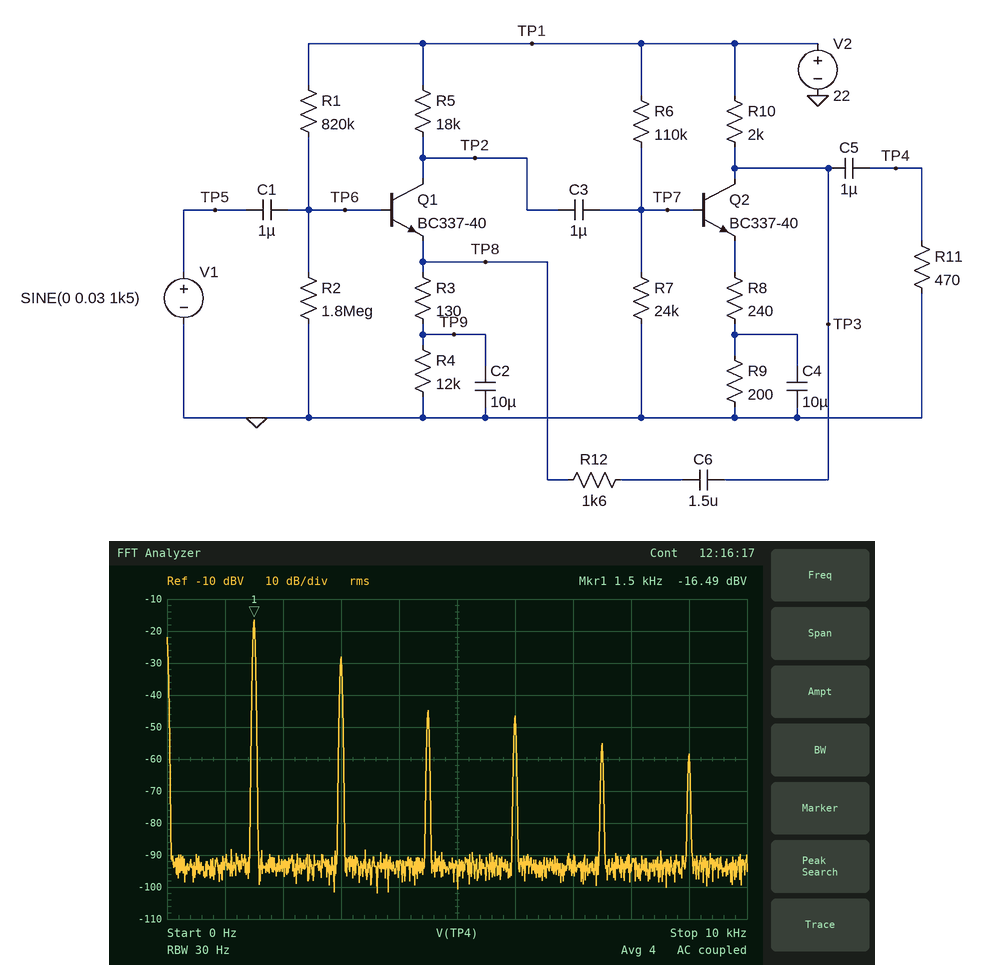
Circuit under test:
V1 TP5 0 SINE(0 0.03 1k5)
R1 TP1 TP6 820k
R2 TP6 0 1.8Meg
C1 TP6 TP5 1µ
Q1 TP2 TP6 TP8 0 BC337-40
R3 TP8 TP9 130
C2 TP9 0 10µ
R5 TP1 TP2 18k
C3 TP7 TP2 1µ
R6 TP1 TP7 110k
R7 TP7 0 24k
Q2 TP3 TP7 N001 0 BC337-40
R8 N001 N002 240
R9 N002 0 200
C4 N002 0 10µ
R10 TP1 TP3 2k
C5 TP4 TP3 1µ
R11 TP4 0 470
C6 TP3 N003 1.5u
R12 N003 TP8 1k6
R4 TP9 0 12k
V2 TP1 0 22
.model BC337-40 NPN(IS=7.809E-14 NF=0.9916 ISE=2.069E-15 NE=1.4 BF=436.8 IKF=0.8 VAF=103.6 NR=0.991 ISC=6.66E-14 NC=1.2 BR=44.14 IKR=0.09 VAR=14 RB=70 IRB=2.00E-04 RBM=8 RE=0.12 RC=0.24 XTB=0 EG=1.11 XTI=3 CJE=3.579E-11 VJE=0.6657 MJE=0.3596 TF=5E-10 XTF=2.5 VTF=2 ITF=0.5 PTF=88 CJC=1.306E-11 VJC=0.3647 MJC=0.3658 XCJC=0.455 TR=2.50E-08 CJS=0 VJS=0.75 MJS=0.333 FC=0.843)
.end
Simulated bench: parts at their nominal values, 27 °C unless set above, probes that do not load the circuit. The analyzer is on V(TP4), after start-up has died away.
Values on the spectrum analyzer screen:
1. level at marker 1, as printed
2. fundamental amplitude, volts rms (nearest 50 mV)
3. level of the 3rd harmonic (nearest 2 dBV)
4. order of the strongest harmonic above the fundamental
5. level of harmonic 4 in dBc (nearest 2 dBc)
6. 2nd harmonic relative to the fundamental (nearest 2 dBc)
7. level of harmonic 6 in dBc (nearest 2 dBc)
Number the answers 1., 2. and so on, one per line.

1. -16.49 dBV
2. 150 mV
3. -44 dBV
4. 2
5. -30 dBc
6. -12 dBc
7. -42 dBc
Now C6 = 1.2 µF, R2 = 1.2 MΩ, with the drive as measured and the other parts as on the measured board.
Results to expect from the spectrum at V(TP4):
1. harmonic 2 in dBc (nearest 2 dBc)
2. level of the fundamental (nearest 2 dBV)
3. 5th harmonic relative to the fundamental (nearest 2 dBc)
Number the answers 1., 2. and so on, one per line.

1. -14 dBc
2. -16 dBV
3. -36 dBc
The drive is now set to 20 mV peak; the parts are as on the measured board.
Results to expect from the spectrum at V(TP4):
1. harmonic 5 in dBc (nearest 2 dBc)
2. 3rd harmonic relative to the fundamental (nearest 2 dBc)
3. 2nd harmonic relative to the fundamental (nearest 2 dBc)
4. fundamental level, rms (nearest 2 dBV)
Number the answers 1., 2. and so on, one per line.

1. -40 dBc
2. -34 dBc
3. -10 dBc
4. -22 dBV
